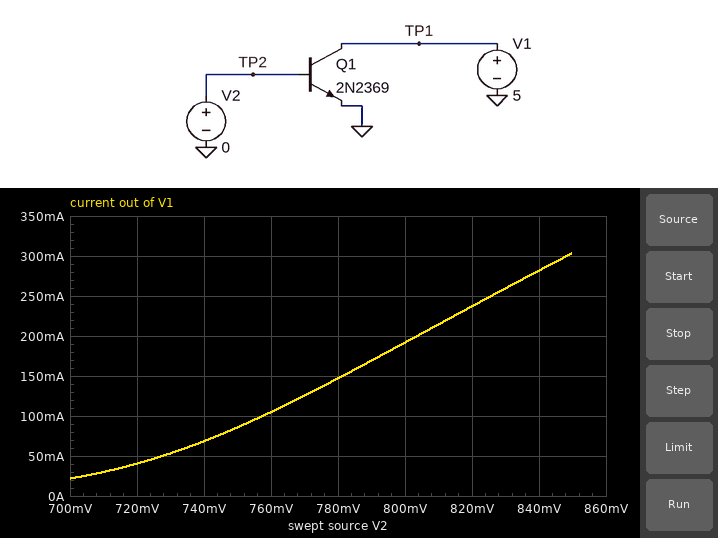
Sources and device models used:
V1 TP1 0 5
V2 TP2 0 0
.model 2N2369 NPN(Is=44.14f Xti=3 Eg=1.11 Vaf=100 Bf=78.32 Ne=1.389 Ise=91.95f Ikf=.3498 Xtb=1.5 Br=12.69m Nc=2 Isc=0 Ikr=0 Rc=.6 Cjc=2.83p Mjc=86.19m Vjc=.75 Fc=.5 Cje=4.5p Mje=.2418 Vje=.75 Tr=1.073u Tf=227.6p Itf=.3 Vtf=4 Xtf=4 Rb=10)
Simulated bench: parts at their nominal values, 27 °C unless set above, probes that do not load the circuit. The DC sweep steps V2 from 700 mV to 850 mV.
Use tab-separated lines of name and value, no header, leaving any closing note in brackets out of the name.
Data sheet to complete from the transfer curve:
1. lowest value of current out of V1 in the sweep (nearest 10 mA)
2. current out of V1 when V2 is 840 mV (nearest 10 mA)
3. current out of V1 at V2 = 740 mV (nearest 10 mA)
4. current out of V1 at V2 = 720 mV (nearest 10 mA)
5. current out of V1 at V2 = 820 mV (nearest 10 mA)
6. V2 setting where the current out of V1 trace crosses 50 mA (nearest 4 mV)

lowest value of current out of V1 in the sweep	20 mA
current out of V1 when V2 is 840 mV	280 mA
current out of V1 at V2 = 740 mV	70 mA
current out of V1 at V2 = 720 mV	40 mA
current out of V1 at V2 = 820 mV	240 mA
V2 setting where the current out of V1 trace crosses 50 mA	728 mV
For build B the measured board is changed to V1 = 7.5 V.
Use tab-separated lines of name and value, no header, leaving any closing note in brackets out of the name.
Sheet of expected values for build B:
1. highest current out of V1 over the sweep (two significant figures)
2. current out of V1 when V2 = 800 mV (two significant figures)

highest current out of V1 over the sweep	310 mA
current out of V1 when V2 = 800 mV	200 mA
